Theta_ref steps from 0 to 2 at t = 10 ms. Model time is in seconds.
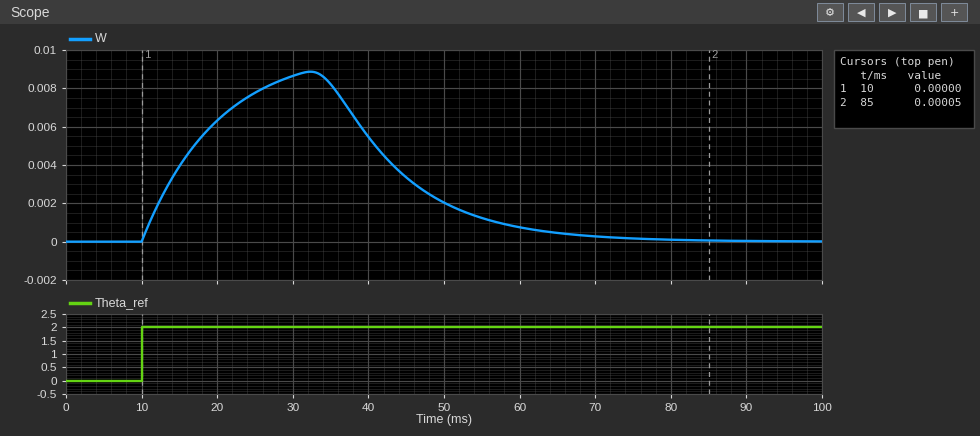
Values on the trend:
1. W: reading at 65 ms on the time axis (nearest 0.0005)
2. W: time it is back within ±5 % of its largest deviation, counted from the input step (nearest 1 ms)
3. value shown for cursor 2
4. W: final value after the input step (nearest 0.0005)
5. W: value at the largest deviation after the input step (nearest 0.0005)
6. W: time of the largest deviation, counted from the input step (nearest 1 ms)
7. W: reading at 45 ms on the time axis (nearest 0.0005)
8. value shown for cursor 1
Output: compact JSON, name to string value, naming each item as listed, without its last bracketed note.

{"W: reading at 65 ms on the time axis": "0.0005", "W: time it is back within ±5 % of its largest deviation, counted from the input step": "55 ms", "value shown for cursor 2": "0.00005", "W: final value after the input step": "0.0000", "W: value at the largest deviation after the input step": "0.0090", "W: time of the largest deviation, counted from the input step": "22 ms", "W: reading at 45 ms on the time axis": "0.0035", "value shown for cursor 1": "0.00000"}
